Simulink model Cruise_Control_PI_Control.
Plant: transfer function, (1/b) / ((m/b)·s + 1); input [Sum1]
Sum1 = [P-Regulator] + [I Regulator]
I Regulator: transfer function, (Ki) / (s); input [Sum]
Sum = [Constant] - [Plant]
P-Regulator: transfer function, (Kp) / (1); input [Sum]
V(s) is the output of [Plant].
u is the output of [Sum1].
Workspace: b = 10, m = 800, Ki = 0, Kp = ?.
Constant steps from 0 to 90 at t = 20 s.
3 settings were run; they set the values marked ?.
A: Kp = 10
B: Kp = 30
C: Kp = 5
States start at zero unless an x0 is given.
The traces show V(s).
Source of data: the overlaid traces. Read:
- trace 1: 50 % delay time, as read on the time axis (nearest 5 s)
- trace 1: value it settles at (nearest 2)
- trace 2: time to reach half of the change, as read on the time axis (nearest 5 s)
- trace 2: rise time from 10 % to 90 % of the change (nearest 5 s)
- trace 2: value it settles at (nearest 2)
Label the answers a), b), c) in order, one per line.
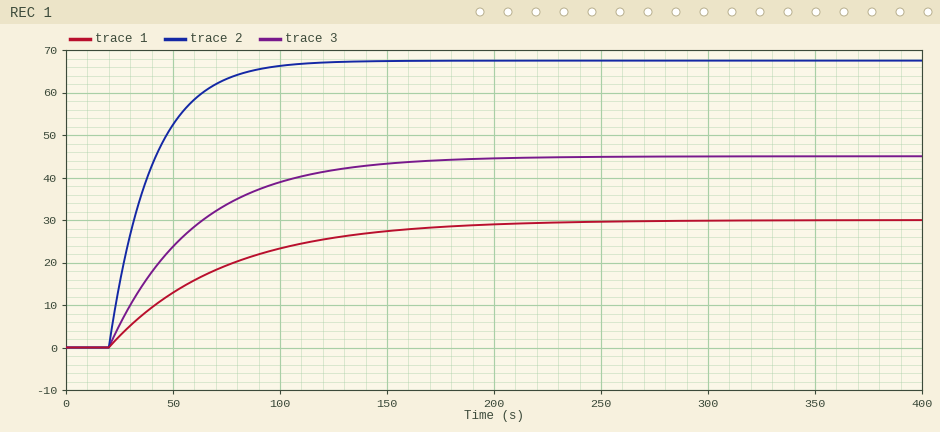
a) 55 s
b) 30
c) 35 s
d) 45 s
e) 68
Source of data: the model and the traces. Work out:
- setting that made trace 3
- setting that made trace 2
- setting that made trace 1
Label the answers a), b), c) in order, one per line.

a) A
b) B
c) C
